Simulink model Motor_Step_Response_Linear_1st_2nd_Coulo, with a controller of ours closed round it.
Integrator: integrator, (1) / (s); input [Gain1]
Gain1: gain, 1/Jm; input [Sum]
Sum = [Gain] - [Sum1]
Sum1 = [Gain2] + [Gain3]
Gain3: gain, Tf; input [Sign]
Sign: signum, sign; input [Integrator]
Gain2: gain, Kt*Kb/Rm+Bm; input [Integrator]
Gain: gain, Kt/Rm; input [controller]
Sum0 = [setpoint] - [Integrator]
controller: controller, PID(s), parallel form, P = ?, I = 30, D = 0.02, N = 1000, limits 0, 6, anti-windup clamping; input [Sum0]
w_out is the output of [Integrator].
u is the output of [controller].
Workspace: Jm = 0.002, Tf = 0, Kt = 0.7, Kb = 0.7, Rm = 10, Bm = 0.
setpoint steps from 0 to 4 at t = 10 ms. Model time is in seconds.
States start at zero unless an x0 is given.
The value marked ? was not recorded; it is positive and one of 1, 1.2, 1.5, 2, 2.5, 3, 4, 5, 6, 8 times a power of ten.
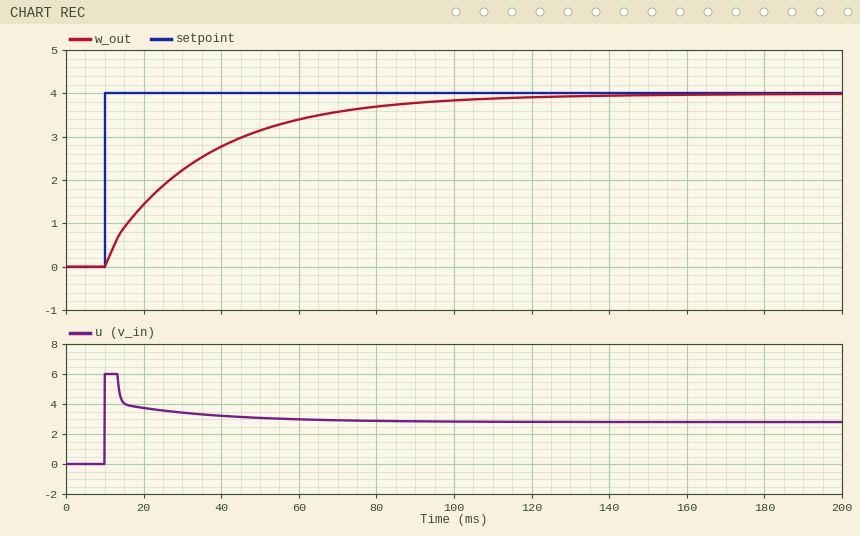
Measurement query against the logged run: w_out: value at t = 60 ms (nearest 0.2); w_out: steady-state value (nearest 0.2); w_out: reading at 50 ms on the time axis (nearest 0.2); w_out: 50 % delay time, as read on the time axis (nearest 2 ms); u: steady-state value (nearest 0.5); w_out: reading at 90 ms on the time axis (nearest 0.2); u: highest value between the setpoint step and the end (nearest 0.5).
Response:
3.4
4.0
3.2
26 ms
3.0
3.8
6.0
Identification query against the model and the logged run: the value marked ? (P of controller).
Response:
2
